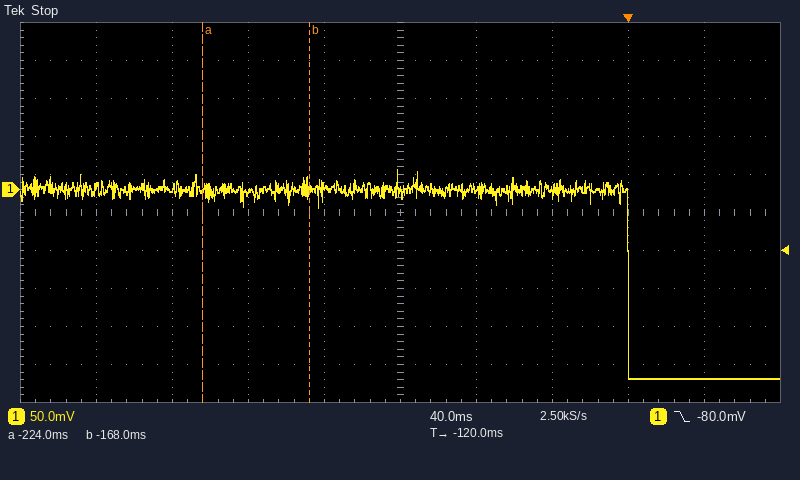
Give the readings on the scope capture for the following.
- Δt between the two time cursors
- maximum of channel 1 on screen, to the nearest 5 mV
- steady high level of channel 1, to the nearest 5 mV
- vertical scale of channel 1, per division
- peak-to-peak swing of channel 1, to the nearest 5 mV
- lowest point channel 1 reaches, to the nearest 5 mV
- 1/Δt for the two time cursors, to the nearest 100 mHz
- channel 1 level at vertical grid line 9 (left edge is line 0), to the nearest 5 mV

56 ms
25 mV
0 mV
50 mV
275 mV
-250 mV
17.9 Hz
-250 mV
